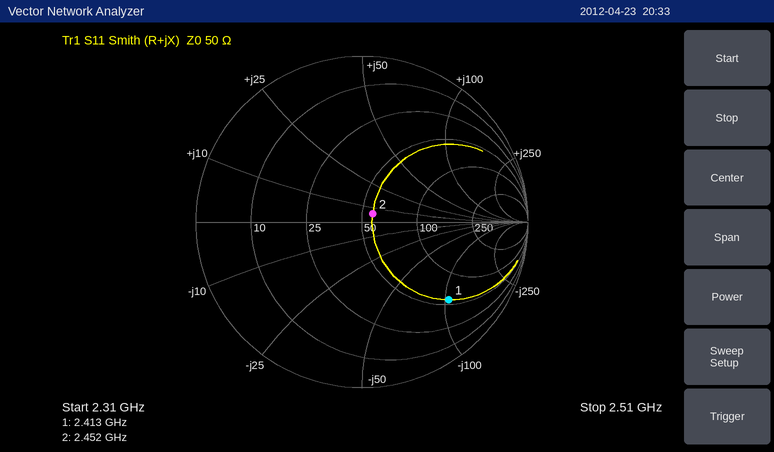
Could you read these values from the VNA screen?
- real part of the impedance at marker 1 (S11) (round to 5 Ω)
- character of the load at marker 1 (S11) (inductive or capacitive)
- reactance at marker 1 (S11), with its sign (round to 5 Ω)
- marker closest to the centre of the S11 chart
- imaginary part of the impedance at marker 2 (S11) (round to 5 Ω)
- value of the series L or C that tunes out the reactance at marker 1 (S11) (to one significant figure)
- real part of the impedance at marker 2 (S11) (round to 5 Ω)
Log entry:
55 Ω
capacitive
-105 Ω
marker 2
+5 Ω
7 nH
55 Ω
